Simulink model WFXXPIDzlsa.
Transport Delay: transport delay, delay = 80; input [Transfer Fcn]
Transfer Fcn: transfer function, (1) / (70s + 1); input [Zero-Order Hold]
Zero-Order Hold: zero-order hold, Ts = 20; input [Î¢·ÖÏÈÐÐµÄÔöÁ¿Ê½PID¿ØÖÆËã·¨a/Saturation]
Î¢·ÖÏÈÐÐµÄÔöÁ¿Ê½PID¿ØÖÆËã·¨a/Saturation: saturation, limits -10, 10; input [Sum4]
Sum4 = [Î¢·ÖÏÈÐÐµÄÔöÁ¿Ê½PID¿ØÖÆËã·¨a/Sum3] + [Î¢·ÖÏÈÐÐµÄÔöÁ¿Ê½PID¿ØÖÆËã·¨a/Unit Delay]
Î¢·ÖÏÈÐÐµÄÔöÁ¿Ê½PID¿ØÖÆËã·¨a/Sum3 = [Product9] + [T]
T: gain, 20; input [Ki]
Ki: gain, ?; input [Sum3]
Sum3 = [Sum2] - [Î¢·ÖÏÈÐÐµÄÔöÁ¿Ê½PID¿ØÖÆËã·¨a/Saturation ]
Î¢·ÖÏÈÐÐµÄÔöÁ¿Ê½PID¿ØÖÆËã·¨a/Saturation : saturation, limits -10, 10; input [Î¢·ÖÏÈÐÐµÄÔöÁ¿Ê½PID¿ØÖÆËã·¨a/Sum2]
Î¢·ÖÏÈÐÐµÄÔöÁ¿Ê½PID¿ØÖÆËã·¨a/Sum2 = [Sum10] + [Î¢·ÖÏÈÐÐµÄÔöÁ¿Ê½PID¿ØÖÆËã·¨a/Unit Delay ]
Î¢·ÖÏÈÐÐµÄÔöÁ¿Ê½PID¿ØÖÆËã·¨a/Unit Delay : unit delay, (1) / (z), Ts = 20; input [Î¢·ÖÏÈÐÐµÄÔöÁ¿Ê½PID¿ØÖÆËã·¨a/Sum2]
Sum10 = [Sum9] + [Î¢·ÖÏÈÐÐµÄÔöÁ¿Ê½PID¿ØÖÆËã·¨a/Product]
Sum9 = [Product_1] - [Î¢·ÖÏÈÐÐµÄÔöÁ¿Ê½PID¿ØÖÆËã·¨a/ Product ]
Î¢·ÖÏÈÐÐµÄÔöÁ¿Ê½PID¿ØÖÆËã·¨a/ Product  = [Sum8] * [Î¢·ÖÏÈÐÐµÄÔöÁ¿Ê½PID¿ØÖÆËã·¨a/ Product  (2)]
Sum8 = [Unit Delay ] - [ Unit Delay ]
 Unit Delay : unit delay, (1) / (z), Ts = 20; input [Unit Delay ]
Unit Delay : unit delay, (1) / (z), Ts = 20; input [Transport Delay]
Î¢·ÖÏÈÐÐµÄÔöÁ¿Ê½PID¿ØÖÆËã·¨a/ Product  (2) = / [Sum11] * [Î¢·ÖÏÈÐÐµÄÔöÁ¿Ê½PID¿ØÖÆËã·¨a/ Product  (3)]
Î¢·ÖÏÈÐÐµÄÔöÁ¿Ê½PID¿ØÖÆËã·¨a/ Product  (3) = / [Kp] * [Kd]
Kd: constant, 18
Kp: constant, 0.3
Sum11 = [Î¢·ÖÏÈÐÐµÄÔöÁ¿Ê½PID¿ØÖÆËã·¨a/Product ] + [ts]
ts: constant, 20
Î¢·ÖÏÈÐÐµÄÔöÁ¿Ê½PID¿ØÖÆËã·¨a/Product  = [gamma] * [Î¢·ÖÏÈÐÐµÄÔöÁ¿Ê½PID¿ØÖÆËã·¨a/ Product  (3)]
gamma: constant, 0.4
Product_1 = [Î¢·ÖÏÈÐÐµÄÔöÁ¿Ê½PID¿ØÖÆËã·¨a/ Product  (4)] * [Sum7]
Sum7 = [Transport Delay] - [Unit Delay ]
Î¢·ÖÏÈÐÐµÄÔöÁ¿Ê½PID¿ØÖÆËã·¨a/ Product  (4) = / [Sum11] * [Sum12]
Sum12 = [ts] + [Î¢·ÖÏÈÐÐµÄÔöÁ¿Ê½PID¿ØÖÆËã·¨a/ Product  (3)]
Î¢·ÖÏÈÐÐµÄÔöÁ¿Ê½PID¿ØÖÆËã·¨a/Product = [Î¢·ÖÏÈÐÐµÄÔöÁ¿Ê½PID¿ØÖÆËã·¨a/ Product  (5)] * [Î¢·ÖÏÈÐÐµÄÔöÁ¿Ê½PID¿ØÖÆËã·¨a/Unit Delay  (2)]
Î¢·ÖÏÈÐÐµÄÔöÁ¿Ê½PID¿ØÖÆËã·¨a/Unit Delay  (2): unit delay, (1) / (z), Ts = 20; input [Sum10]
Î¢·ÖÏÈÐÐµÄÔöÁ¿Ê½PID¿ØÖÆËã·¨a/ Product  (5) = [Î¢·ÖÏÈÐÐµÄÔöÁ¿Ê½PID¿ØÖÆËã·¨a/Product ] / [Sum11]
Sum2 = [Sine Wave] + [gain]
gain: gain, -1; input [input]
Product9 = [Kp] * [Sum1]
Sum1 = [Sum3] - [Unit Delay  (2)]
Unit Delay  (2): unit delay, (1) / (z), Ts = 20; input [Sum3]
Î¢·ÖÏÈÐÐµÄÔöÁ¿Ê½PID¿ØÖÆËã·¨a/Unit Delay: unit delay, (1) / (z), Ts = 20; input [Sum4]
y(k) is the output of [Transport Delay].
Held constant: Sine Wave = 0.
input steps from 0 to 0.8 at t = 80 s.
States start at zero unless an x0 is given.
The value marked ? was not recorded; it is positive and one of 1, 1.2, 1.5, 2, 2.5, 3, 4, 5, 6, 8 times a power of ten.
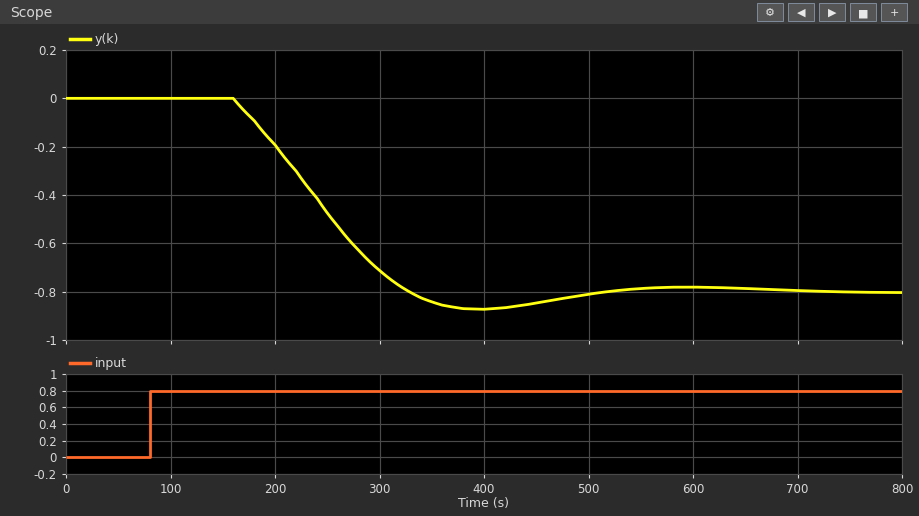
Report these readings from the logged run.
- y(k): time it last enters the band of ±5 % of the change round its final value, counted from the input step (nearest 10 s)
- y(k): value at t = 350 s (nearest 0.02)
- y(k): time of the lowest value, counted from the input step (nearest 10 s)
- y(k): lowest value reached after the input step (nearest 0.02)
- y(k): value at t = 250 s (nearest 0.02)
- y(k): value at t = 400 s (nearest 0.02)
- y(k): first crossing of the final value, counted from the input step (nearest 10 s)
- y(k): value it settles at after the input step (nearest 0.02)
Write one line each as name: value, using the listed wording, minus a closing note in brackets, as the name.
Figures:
y(k): time it last enters the band of ±5 % of the change round its final value, counted from the input step: 380 s
y(k): value at t = 350 s: -0.84
y(k): time of the lowest value, counted from the input step: 320 s
y(k): lowest value reached after the input step: -0.88
y(k): value at t = 250 s: -0.48
y(k): value at t = 400 s: -0.88
y(k): first crossing of the final value, counted from the input step: 250 s
y(k): value it settles at after the input step: -0.80
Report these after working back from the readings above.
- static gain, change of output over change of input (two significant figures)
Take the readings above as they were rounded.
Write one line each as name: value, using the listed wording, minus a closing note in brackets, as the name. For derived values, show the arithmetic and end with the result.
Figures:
static gain, change of output over change of input: (-0.8 - 0) / (0.8 - 0) = -1.0
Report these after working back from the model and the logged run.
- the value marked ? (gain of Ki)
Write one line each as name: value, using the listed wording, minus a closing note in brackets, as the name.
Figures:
the value marked ?: 0.008
